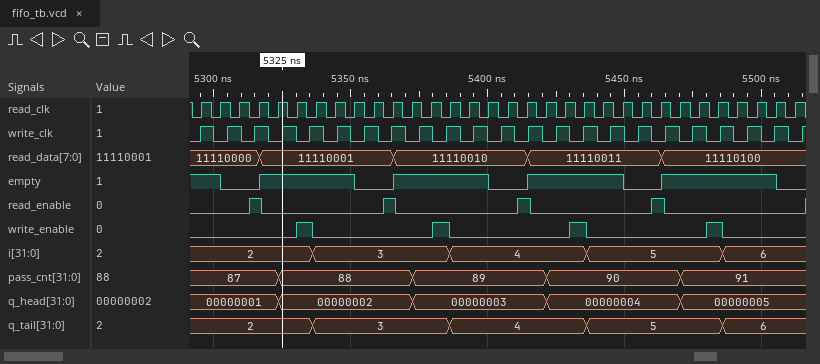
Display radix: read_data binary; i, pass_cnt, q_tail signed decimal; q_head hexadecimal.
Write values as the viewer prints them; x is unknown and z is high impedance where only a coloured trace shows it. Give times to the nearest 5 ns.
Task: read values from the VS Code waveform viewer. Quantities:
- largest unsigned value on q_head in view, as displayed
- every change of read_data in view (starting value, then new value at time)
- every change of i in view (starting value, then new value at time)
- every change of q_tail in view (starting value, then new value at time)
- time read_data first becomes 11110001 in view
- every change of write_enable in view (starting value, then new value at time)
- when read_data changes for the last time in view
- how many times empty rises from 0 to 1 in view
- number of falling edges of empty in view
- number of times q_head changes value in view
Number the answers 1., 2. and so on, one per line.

1. 00000005
2. 11110000, 11110001 at 5315 ns, 11110010 at 5365 ns, 11110011 at 5415 ns, 11110100 at 5465 ns
3. 2, 3 at 5335 ns, 4 at 5385 ns, 5 at 5435 ns, 6 at 5485 ns
4. 2, 3 at 5335 ns, 4 at 5385 ns, 5 at 5435 ns, 6 at 5485 ns
5. 5315 ns
6. 0, 1 at 5330 ns, 0 at 5335 ns, 1 at 5380 ns, 0 at 5385 ns, 1 at 5430 ns, 0 at 5435 ns, 1 at 5480 ns, 0 at 5485 ns
7. 5465 ns
8. 4
9. 5
10. 4
